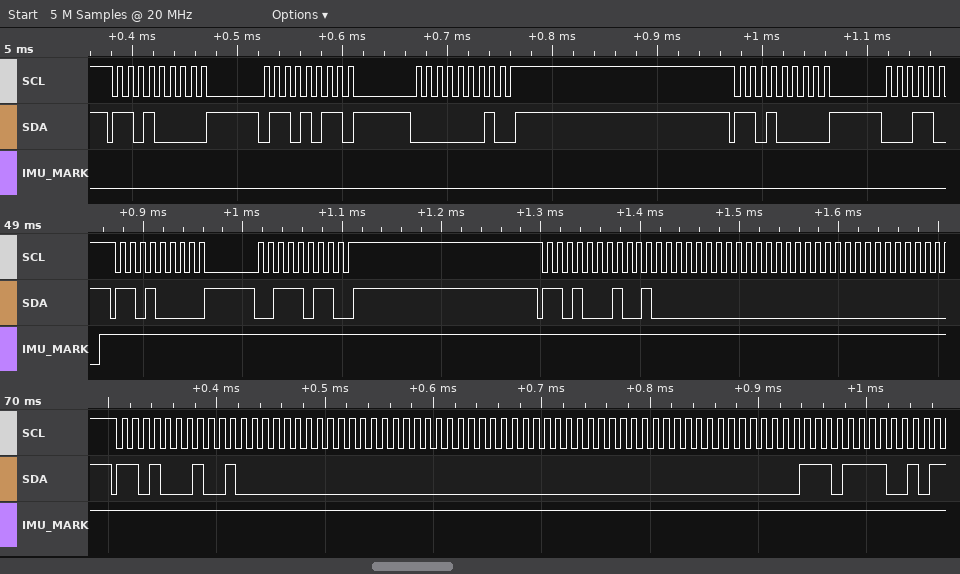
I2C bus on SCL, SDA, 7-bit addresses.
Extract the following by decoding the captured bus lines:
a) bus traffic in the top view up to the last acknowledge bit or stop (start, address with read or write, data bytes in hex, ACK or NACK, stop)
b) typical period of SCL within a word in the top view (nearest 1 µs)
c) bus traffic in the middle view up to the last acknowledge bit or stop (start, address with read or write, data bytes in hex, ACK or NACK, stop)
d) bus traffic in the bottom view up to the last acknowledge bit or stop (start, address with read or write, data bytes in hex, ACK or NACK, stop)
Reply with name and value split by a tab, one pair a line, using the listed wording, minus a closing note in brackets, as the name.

bus traffic in the top view up to the last acknowledge bit or stop	start, address 68 write ACK, 6B ACK, 01 ACK, stop, start, address 68 write ACK
typical period of SCL within a word in the top view	10 µs
bus traffic in the middle view up to the last acknowledge bit or stop	start, address 68 write ACK, 3B ACK, stop, start, address 68 read ACK, 40 ACK, 00 ACK, 00 ACK
bus traffic in the bottom view up to the last acknowledge bit or stop	start, address 68 read ACK, 40 ACK, 00 ACK, 00 ACK, 00 ACK, 00 ACK, 00 ACK, EF ACK
